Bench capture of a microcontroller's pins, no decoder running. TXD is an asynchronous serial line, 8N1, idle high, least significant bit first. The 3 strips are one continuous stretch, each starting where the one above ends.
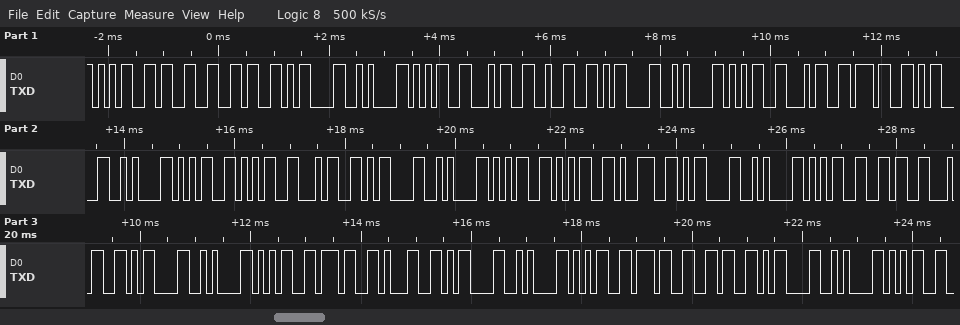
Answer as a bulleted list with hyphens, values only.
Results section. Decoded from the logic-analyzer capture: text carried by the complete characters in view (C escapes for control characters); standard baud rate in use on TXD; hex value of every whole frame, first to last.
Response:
- "536\r\n542\r\n547\r\n554\r\n559\r\n564\r\n571\r\n576\r\n5"
- 9600 baud
- 35 33 36 0D 0A 35 34 32 0D 0A 35 34 37 0D 0A 35 35 34 0D 0A 35 35 39 0D 0A 35 36 34 0D 0A 35 37 31 0D 0A 35 37 36 0D 0A 35
